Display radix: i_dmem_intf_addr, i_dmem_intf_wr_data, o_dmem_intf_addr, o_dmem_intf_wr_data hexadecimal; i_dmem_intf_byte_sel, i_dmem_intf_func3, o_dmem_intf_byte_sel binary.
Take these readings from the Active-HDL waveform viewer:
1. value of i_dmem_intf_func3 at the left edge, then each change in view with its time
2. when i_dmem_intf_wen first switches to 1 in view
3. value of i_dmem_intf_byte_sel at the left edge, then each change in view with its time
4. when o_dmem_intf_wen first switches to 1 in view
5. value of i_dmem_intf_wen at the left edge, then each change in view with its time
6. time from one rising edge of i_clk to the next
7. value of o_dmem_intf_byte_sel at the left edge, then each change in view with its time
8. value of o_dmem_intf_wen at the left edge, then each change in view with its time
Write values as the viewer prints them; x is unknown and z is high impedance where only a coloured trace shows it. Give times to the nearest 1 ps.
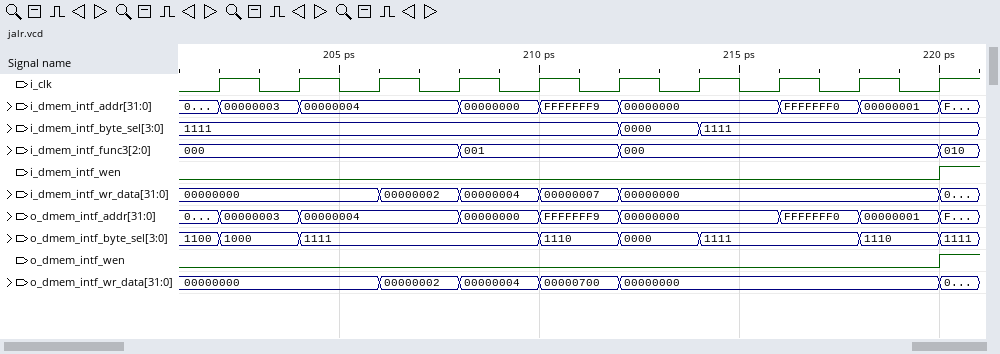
000, 001 at 208 ps, 000 at 212 ps, 010 at 220 ps
220 ps
1111, 0000 at 212 ps, 1111 at 214 ps
220 ps
0, 1 at 220 ps
2 ps
1100, 1000 at 202 ps, 1111 at 204 ps, 1110 at 210 ps, 0000 at 212 ps, 1111 at 214 ps, 1110 at 218 ps, 1111 at 220 ps
0, 1 at 220 ps
